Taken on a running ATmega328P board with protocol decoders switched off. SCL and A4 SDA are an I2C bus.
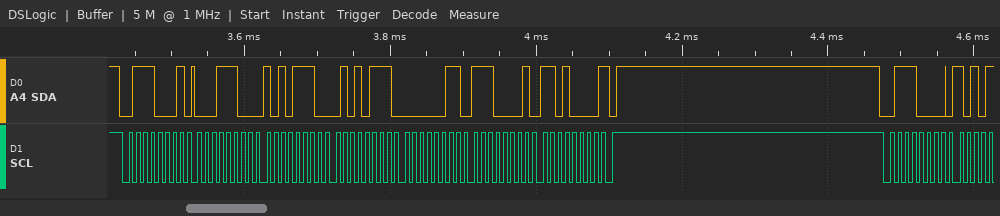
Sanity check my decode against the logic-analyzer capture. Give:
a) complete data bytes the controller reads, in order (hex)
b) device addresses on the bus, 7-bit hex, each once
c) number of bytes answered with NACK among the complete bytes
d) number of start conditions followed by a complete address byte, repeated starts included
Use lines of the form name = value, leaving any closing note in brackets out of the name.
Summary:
complete data bytes the controller reads, in order = 1C AE 57 03 E1 D0
device addresses on the bus, 7-bit hex, each once = 0x38
number of bytes answered with NACK among the complete bytes = 1
number of start conditions followed by a complete address byte, repeated starts included = 2
